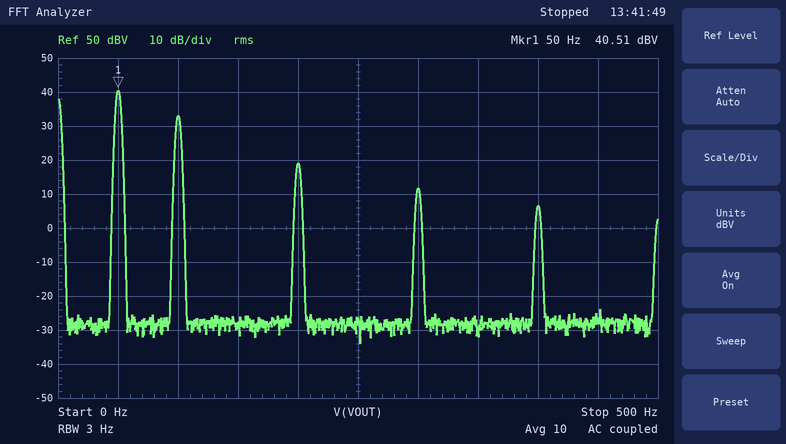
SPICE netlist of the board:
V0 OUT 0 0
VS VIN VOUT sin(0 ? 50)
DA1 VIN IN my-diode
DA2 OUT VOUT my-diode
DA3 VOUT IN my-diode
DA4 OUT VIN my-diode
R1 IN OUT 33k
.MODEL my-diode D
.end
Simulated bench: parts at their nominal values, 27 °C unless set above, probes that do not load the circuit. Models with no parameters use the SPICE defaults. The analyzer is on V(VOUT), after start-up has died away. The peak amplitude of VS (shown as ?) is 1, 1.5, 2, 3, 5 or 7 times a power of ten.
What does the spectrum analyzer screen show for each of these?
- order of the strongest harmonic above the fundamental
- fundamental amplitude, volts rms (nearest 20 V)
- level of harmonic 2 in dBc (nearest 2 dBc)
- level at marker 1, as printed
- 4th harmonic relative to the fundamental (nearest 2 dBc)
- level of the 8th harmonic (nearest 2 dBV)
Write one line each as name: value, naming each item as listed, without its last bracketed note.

order of the strongest harmonic above the fundamental: 2
fundamental amplitude, volts rms: 100 V
level of harmonic 2 in dBc: -8 dBc
level at marker 1, as printed: 40.51 dBV
4th harmonic relative to the fundamental: -22 dBc
level of the 8th harmonic: 6 dBV
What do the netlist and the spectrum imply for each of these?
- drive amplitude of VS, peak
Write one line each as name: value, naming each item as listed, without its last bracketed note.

drive amplitude of VS, peak: 300 V
